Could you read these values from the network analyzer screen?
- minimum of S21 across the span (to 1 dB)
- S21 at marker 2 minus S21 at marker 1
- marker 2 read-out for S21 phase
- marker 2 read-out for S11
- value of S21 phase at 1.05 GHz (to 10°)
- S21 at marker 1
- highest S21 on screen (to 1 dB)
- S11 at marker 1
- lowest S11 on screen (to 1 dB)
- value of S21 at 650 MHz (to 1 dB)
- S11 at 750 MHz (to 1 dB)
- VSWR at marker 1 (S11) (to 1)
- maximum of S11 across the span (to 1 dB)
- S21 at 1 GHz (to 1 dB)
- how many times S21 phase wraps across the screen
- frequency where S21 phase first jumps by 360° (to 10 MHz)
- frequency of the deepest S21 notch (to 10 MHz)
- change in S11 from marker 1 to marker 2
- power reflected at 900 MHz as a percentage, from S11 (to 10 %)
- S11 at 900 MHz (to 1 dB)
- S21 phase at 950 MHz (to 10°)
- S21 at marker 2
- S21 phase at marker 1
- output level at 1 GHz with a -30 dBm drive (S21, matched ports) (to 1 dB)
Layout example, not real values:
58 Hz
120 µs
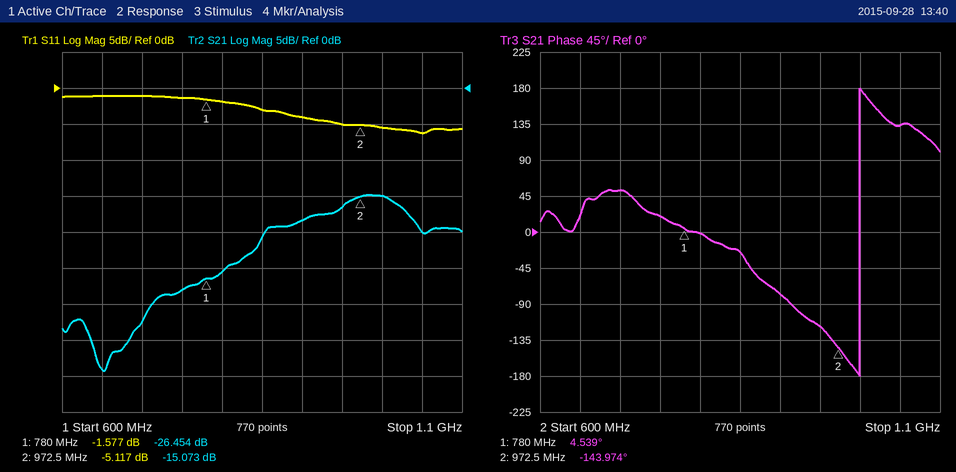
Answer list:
-39 dB
11.381 dB
-143.974°
-5.117 dB
130°
-26.454 dB
-15 dB
-1.577 dB
-6 dB
-39 dB
-1 dB
11
-1 dB
-15 dB
1
1.00 GHz
650 MHz
-3.540 dB
40 %
-4 dB
-120°
-15.073 dB
4.539°
-45 dBm
